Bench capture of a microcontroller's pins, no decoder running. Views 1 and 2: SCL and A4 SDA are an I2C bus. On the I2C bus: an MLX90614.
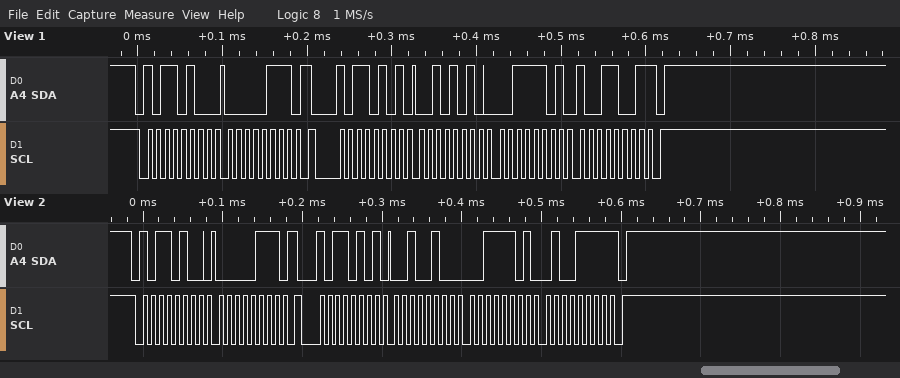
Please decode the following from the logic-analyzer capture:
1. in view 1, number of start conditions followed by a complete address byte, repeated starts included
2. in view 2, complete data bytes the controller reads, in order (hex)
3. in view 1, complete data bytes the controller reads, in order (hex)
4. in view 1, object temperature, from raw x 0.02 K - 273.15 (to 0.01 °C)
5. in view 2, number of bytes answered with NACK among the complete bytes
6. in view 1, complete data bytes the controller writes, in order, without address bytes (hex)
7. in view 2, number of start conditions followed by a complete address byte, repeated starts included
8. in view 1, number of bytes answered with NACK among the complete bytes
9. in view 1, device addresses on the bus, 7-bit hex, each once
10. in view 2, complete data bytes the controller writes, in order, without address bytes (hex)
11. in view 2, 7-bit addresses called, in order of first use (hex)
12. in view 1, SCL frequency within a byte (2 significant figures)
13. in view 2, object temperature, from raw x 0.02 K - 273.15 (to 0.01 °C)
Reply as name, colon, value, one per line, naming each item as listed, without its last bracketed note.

in view 1, number of start conditions followed by a complete address byte, repeated starts included: 2
in view 2, complete data bytes the controller reads, in order: 24 3D 4F
in view 1, complete data bytes the controller reads, in order: 2A 3D 99
in view 1, object temperature, from raw x 0.02 K - 273.15: 40.01 °C
in view 2, number of bytes answered with NACK among the complete bytes: 1
in view 1, complete data bytes the controller writes, in order, without address bytes: 07
in view 2, number of start conditions followed by a complete address byte, repeated starts included: 2
in view 1, number of bytes answered with NACK among the complete bytes: 1
in view 1, device addresses on the bus, 7-bit hex, each once: 0x5A
in view 2, complete data bytes the controller writes, in order, without address bytes: 07
in view 2, 7-bit addresses called, in order of first use: 0x5A
in view 1, SCL frequency within a byte: 100 kHz
in view 2, object temperature, from raw x 0.02 K - 273.15: 39.89 °C
